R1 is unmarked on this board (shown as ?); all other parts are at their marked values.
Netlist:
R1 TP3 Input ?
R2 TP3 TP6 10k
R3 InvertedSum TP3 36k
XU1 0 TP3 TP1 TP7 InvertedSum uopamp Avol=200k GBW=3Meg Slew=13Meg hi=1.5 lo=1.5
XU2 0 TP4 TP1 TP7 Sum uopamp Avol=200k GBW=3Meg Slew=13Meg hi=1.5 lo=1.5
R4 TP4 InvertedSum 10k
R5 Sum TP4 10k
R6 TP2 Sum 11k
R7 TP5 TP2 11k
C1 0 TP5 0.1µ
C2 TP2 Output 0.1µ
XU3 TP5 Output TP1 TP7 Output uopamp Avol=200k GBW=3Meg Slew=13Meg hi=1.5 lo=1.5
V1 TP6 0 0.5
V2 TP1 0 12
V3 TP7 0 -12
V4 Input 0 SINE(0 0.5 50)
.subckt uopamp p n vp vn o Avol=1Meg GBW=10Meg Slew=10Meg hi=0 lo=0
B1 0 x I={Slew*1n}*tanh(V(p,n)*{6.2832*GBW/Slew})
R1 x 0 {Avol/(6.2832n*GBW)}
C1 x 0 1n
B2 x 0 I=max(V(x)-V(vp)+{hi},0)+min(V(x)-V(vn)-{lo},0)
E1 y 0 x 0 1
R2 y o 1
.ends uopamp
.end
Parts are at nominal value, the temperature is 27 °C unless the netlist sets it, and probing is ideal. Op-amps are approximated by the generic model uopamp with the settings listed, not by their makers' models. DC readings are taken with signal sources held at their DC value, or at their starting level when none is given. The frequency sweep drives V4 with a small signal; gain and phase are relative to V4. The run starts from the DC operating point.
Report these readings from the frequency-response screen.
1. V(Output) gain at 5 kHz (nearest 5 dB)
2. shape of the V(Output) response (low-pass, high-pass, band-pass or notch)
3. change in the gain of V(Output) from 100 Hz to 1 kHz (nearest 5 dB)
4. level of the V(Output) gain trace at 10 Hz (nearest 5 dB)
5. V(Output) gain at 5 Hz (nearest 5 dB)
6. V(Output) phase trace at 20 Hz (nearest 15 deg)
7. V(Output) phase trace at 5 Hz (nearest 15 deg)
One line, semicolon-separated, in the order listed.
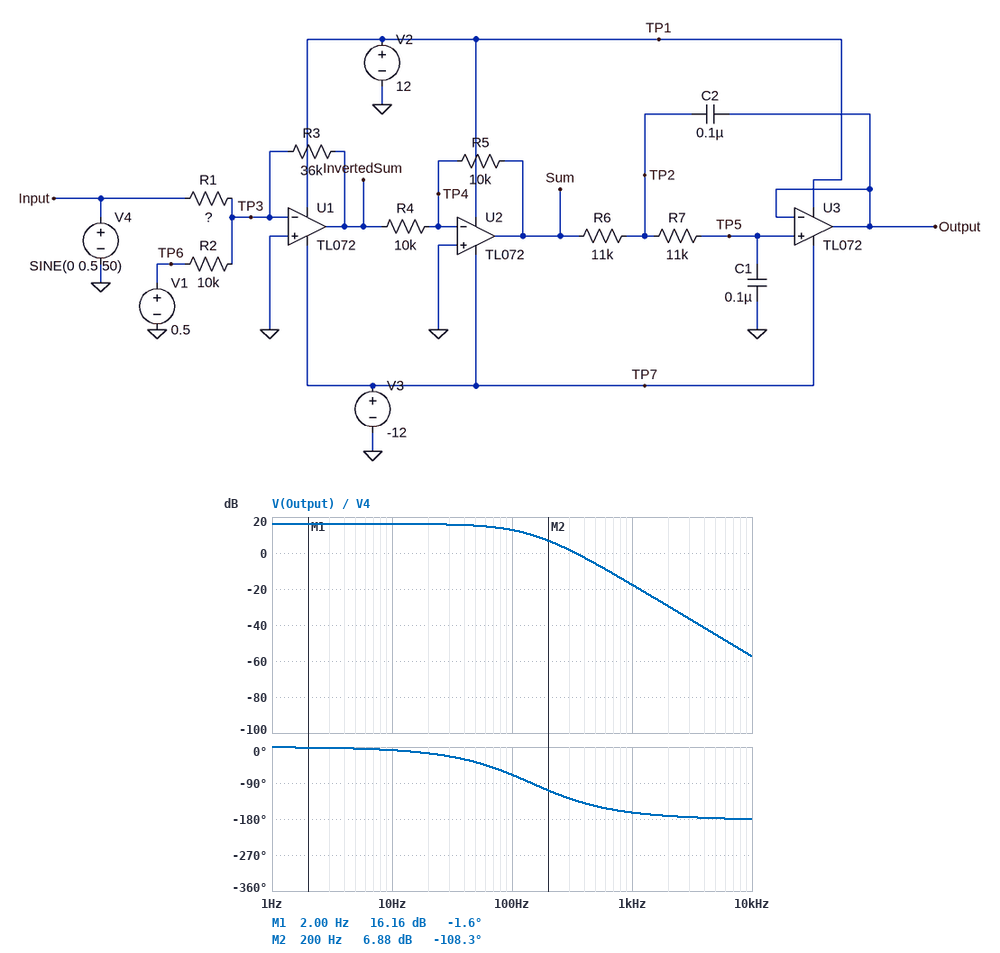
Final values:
-45 dB; low-pass; -30 dB; 15 dB; 15 dB; -15 deg; 0 deg
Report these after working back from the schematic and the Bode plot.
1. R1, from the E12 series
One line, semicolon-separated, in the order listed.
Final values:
5.6 kΩ
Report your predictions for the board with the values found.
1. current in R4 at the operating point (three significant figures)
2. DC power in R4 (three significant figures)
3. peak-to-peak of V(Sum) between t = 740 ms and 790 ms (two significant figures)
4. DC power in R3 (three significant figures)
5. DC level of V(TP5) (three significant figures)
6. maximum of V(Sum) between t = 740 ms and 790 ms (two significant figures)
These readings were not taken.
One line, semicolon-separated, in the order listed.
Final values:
180 µA; 324 µW; 6.4 V; 90.0 µW; 1.80 V; 5.0 V
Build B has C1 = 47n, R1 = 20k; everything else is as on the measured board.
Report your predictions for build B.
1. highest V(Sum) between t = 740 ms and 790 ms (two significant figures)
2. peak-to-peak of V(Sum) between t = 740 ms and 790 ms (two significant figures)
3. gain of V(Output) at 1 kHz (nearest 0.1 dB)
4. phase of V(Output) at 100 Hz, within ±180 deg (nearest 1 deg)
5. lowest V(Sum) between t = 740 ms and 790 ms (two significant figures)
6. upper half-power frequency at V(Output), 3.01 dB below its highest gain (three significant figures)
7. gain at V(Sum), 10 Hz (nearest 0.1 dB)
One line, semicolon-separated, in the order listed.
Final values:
2.7 V; 1.8 V; -21.9 dB; -40 deg; 900 mV; 217 Hz; 5.1 dB
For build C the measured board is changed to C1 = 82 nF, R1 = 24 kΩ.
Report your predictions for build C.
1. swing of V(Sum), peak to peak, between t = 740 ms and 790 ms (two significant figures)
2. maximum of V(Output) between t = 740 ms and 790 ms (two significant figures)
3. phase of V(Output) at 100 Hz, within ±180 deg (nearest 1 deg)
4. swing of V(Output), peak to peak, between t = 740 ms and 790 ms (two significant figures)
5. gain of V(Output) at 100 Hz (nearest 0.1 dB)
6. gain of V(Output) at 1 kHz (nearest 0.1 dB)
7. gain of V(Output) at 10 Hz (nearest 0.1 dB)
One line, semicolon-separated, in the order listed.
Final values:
1.5 V; 2.5 V; -62 deg; 1.4 V; 1.3 dB; -28.5 dB; 3.5 dB
